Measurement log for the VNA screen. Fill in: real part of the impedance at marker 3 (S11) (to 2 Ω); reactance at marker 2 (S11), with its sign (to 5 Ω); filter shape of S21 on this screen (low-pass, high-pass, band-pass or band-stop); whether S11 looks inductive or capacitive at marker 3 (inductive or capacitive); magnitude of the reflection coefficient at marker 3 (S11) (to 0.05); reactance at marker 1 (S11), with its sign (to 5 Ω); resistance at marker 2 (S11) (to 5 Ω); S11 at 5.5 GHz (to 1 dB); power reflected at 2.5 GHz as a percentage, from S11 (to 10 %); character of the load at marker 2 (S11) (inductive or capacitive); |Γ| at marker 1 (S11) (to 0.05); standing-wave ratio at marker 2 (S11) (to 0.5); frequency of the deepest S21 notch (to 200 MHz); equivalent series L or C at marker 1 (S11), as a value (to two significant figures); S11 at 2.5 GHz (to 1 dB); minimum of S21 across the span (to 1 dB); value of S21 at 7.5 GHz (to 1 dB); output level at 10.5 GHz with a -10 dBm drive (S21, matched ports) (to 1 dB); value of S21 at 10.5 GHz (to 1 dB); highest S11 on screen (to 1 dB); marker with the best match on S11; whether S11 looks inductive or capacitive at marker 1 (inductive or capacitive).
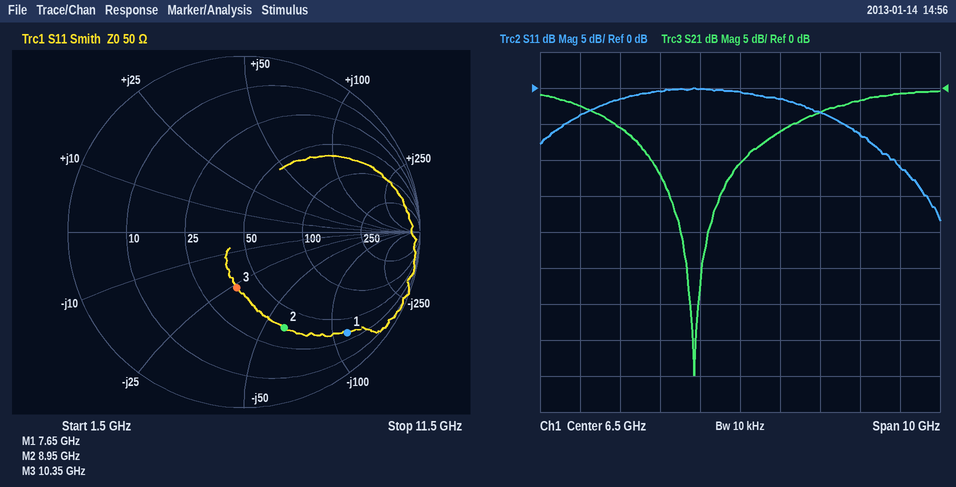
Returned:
38 Ω
-60 Ω
band-stop
capacitive
0.30
-115 Ω
35 Ω
0 dB
40 %
capacitive
0.80
4.0
5.4 GHz
180 fF
-4 dB
-40 dB
-6 dB
-11 dBm
-1 dB
0 dB
marker 3
capacitive
